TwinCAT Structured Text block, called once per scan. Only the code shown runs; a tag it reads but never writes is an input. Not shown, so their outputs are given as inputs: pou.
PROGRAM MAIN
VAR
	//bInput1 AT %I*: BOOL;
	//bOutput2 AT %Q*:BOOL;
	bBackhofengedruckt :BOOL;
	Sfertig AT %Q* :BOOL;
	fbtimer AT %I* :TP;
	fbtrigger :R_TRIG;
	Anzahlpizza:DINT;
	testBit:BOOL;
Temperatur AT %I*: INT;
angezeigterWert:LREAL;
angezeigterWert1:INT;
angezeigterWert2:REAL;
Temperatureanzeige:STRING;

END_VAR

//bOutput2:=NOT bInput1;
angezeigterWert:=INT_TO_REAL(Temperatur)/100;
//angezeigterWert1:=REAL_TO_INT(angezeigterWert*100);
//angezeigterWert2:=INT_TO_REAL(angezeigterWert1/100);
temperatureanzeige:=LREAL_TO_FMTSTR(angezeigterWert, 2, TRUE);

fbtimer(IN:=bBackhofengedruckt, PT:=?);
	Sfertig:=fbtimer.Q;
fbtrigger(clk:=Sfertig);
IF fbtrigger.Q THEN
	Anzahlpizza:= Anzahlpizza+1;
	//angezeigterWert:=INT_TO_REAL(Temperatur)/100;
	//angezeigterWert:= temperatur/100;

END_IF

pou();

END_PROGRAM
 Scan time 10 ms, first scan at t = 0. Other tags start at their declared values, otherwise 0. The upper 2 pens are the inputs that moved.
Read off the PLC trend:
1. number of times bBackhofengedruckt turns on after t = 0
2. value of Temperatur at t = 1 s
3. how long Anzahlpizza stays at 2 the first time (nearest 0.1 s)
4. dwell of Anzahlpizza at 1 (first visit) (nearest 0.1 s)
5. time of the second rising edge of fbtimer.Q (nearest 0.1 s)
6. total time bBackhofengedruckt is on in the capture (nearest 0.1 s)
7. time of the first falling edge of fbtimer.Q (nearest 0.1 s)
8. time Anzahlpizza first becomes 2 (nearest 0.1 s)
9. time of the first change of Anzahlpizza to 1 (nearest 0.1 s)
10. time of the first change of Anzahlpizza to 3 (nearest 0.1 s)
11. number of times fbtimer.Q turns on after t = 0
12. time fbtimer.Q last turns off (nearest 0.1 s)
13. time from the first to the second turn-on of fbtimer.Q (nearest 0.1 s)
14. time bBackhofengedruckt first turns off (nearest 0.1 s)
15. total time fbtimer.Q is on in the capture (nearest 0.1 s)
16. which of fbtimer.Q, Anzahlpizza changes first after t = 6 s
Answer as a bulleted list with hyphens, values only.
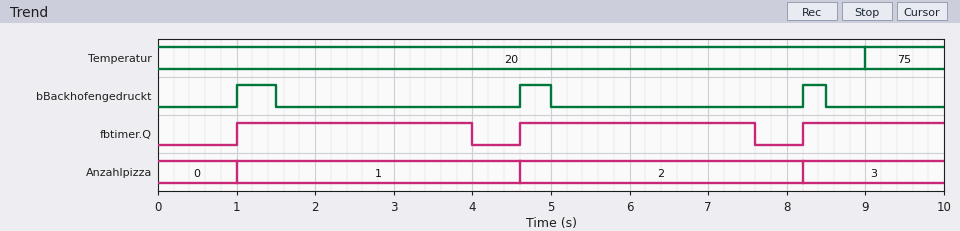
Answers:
- 3
- 20
- 3.6 s
- 3.6 s
- 4.6 s
- 1.2 s
- 4.0 s
- 4.6 s
- 1.0 s
- 8.2 s
- 3
- 7.6 s
- 3.6 s
- 1.5 s
- 7.8 s
- fbtimer.Q
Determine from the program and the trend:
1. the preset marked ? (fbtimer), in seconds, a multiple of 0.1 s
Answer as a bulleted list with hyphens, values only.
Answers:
- 3.0 s
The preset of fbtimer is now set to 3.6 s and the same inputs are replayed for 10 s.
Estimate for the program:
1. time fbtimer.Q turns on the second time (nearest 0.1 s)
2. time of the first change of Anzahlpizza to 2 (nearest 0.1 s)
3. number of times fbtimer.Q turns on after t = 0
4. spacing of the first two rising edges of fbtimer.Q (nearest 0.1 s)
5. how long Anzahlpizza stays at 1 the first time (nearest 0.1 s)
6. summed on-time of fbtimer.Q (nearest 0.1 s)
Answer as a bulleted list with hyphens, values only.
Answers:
- 8.2 s
- 8.2 s
- 2
- 7.2 s
- 7.2 s
- 5.4 s
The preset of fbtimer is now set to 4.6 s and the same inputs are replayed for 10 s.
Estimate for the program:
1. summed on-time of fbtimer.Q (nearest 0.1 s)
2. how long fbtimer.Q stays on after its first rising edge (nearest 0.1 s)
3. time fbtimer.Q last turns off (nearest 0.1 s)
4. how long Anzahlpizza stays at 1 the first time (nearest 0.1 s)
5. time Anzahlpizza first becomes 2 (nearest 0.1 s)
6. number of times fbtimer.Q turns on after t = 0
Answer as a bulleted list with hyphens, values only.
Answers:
- 6.4 s
- 4.6 s
- 5.6 s
- 7.2 s
- 8.2 s
- 2
